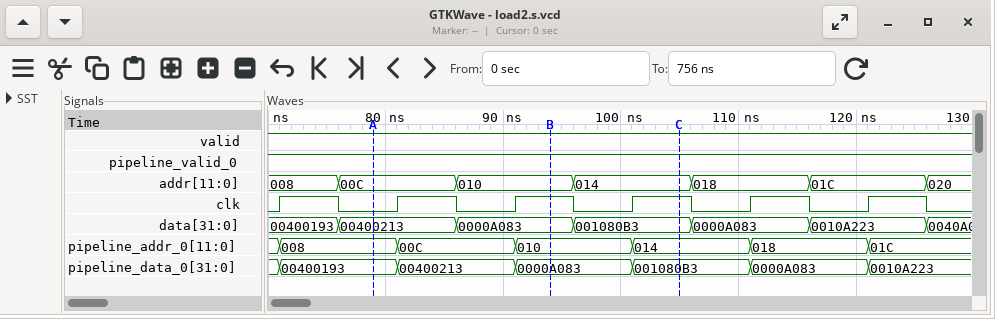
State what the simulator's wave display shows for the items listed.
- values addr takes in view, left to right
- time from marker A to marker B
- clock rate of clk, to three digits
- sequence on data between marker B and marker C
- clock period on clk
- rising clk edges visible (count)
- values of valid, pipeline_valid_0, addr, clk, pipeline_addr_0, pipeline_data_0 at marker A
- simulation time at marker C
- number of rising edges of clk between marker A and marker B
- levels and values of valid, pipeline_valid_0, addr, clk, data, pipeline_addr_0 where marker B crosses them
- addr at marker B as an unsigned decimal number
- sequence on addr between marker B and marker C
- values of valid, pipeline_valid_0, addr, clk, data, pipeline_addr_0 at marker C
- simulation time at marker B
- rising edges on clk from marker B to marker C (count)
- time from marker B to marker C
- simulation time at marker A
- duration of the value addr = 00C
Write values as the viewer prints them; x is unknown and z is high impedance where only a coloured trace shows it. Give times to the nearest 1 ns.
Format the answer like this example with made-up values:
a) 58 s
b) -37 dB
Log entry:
a) 008, 00C, 010, 014, 018, 01C, 020
b) 15 ns
c) 100 MHz
d) 0000A083, 001080B3
e) 10 ns
f) 6
g) valid=1, pipeline_valid_0=1, addr=00C, clk=0, pipeline_addr_0=008, pipeline_data_0=00400193
h) 105 ns
i) 2
j) valid=1, pipeline_valid_0=1, addr=010, clk=1, data=0000A083, pipeline_addr_0=010
k) 16
l) 010, 014
m) valid=1, pipeline_valid_0=1, addr=014, clk=1, data=001080B3, pipeline_addr_0=014
n) 94 ns
o) 1
p) 11 ns
q) 79 ns
r) 10 ns
